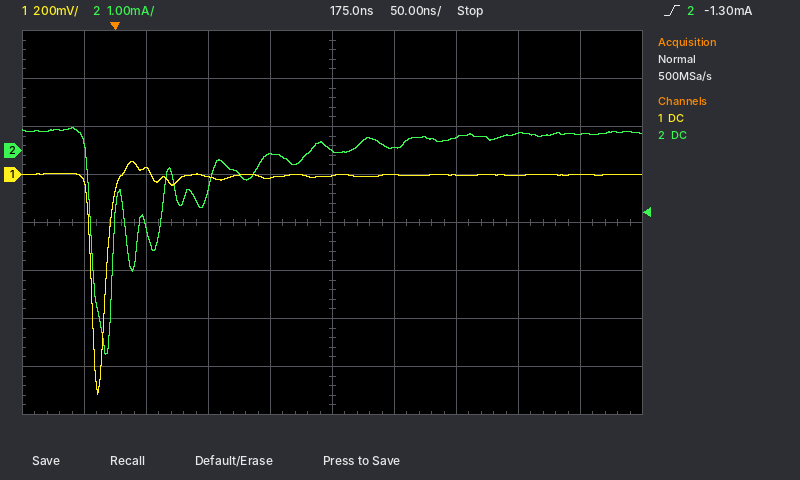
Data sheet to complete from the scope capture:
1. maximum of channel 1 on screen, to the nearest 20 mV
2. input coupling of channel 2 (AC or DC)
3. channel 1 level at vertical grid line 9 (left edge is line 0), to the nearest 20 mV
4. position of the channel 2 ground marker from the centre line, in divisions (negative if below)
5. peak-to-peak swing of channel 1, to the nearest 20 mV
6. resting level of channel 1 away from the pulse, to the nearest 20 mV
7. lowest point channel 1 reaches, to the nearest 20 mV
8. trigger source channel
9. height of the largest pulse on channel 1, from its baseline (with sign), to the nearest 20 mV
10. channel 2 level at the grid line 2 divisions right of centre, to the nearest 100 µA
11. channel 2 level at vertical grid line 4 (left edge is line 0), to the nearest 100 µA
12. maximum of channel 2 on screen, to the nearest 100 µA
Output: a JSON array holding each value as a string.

["60 mV", "DC", "0 mV", "+1.5 div", "980 mV", "0 mV", "-920 mV", "channel 2", "-920 mV", "300 µA", "-100 µA", "500 µA"]
